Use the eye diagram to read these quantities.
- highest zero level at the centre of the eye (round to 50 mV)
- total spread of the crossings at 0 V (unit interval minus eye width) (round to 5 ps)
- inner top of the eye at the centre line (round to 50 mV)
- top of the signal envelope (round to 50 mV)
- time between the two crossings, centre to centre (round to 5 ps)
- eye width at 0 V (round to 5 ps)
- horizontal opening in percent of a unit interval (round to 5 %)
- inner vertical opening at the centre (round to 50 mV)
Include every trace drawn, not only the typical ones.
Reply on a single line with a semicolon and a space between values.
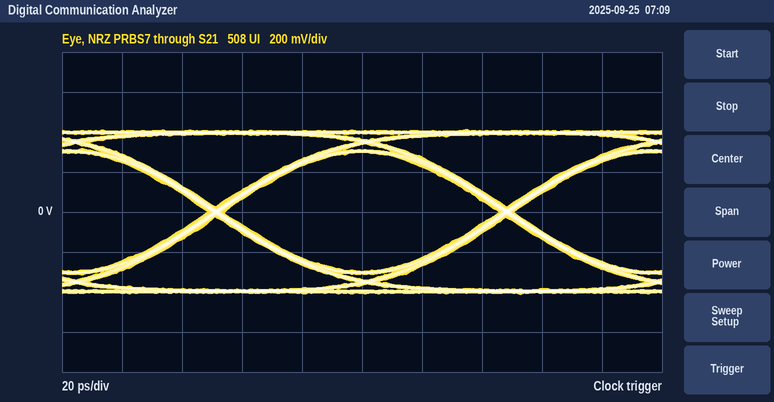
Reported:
-300 mV; 5 ps; 300 mV; 400 mV; 95 ps; 90 ps; 95 %; 600 mV
